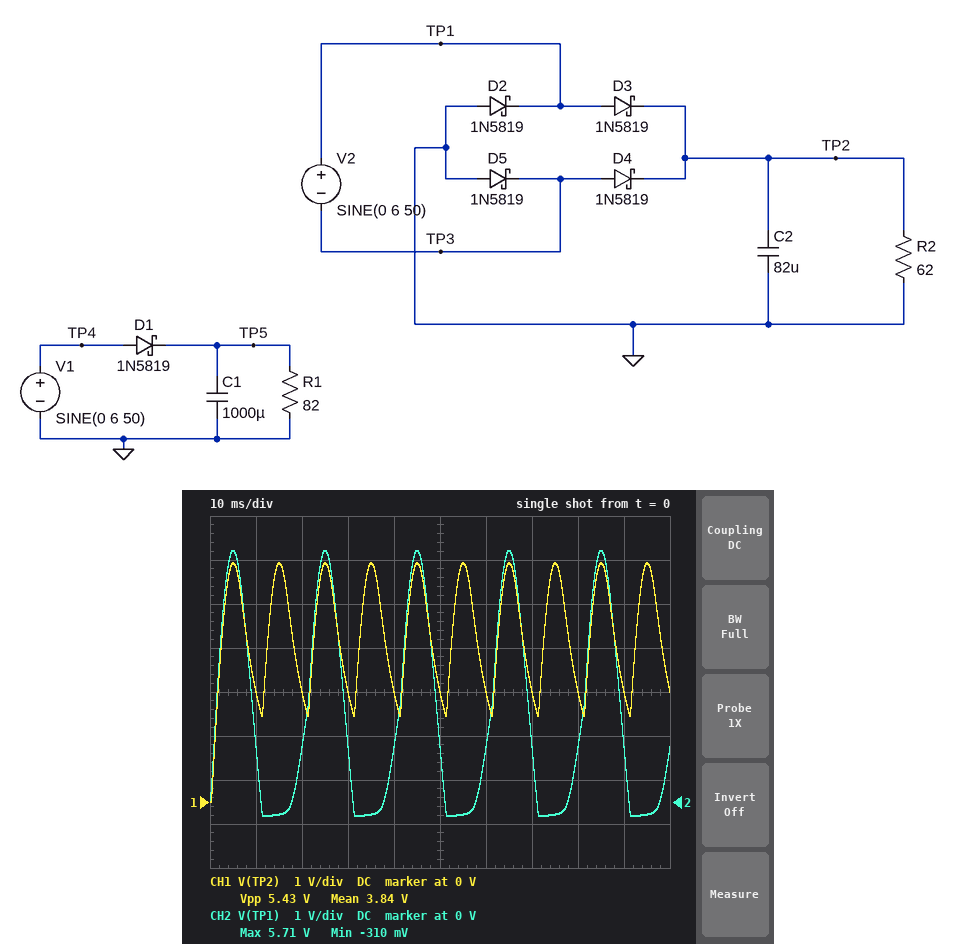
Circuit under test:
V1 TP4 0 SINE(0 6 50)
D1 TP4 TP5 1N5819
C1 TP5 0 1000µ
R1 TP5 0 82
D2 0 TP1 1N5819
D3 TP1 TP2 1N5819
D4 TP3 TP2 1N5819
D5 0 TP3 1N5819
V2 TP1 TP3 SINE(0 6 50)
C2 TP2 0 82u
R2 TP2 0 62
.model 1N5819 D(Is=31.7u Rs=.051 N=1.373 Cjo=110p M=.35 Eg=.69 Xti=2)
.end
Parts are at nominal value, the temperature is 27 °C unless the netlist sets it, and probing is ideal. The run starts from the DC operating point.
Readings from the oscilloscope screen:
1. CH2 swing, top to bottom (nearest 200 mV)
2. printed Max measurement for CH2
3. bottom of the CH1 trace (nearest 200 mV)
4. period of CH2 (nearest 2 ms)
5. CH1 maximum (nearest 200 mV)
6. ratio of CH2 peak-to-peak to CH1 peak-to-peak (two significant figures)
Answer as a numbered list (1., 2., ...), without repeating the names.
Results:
1. 6.0 V
2. 5.71 V
3. 0 V
4. 20 ms
5. 5.4 V
6. 1.1
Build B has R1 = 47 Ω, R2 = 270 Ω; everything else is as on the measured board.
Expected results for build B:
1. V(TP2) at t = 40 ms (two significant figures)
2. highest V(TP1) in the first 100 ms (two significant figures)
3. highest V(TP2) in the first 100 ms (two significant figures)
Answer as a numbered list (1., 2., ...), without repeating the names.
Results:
1. 4.5 V
2. 5.8 V
3. 5.5 V
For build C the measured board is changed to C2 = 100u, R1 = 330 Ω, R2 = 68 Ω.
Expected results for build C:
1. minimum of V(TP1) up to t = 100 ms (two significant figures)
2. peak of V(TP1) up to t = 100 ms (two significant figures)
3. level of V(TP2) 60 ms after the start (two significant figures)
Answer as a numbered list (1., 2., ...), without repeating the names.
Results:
1. -320 mV
2. 5.7 V
3. 3.0 V
